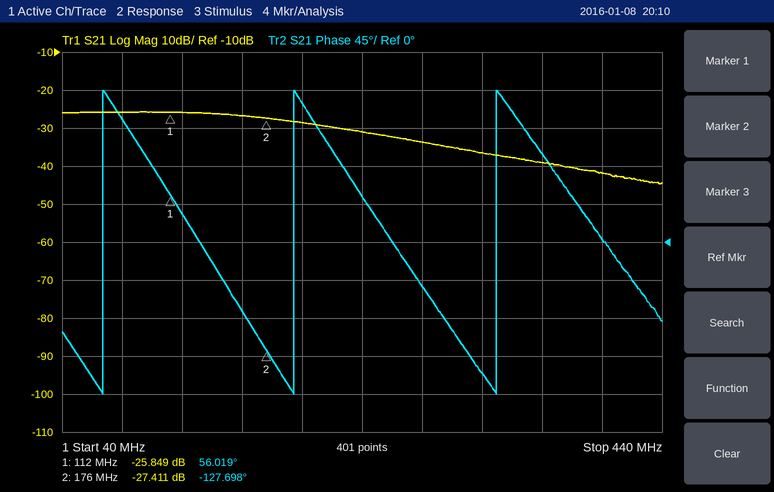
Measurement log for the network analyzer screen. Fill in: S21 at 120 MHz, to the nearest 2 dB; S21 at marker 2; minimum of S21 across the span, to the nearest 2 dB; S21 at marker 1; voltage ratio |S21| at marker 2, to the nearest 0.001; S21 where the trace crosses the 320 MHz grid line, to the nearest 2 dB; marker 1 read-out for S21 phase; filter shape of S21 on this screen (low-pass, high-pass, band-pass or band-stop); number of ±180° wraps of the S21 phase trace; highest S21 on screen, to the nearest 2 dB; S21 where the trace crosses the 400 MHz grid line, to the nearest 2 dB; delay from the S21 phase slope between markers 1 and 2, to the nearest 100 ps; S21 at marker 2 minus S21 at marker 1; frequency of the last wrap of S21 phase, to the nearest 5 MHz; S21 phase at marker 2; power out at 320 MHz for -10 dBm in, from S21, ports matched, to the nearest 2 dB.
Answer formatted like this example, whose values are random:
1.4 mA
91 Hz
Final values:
-26 dB
-27.411 dB
-44 dB
-25.849 dB
0.043
-36 dB
56.019°
low-pass
3
-26 dB
-42 dB
8.0 ns
-1.562 dB
330 MHz
-127.698°
-46 dBm
